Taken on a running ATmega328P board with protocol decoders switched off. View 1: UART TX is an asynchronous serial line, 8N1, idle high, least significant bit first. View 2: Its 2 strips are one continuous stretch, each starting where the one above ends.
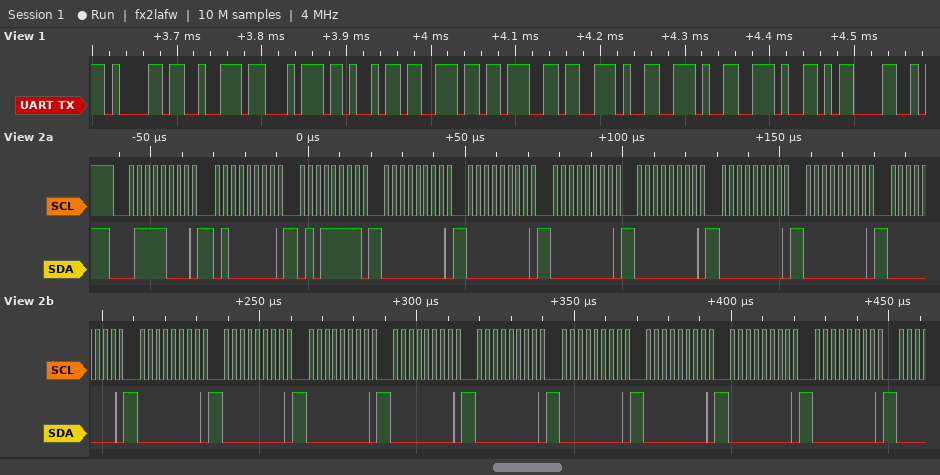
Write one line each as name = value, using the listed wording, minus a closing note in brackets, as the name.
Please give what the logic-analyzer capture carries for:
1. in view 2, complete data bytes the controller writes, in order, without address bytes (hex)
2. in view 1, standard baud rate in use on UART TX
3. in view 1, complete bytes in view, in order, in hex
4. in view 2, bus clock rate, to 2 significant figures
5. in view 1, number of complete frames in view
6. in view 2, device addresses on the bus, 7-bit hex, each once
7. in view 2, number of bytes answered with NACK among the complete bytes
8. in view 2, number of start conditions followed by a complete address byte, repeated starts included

in view 2, complete data bytes the controller writes, in order, without address bytes = 40 5F 00 00 00 00 00 00 00 00 00 00 00 00 00 00 00 00
in view 1, standard baud rate in use on UART TX = 115200 baud
in view 1, complete bytes in view, in order, in hex = 61 72 74 69 6E 67 2E 2E 2E 0D
in view 2, bus clock rate, to 2 significant figures = 400 kHz
in view 1, number of complete frames in view = 10
in view 2, device addresses on the bus, 7-bit hex, each once = 0x3C
in view 2, number of bytes answered with NACK among the complete bytes = 0
in view 2, number of start conditions followed by a complete address byte, repeated starts included = 1
